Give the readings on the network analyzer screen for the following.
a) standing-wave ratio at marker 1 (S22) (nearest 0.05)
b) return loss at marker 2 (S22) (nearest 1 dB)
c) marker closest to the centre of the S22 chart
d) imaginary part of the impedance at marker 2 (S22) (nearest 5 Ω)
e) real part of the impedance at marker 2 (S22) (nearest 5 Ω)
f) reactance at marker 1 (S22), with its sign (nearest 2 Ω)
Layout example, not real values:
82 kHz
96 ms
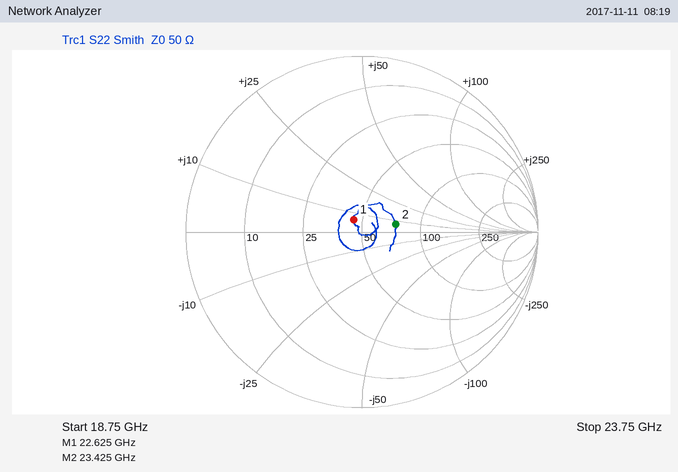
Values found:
1.20
14 dB
marker 1
+5 Ω
75 Ω
+6 Ω
